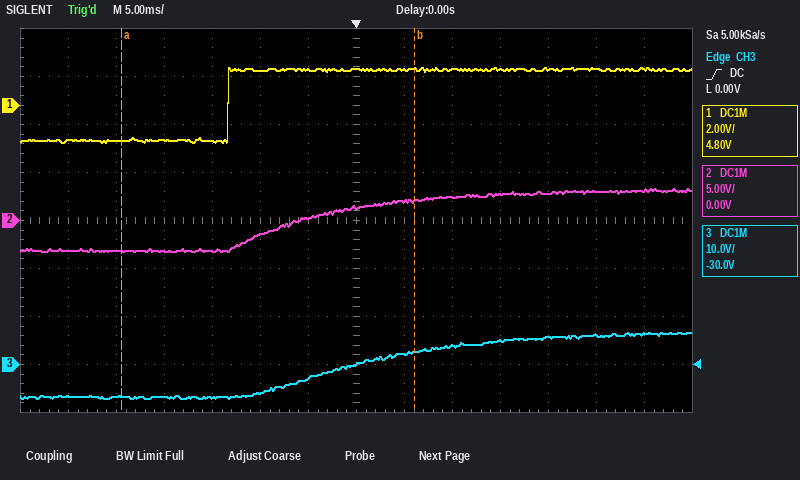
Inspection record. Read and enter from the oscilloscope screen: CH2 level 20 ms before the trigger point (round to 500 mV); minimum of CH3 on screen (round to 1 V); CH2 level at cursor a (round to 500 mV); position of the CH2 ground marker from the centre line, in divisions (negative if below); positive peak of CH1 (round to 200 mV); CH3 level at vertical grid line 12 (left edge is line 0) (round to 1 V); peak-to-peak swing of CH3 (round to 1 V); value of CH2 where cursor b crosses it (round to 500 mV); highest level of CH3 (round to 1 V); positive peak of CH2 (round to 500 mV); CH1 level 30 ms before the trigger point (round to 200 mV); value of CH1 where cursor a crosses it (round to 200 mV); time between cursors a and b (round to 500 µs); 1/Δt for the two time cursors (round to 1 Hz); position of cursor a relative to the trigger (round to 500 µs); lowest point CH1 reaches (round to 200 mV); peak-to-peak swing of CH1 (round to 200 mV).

-3.0 V
-7 V
-3.0 V
0.0 div
1.6 V
6 V
14 V
2.0 V
7 V
3.5 V
-1.4 V
-1.4 V
30.5 ms
33 Hz
-24.5 ms
-1.6 V
3.2 V
